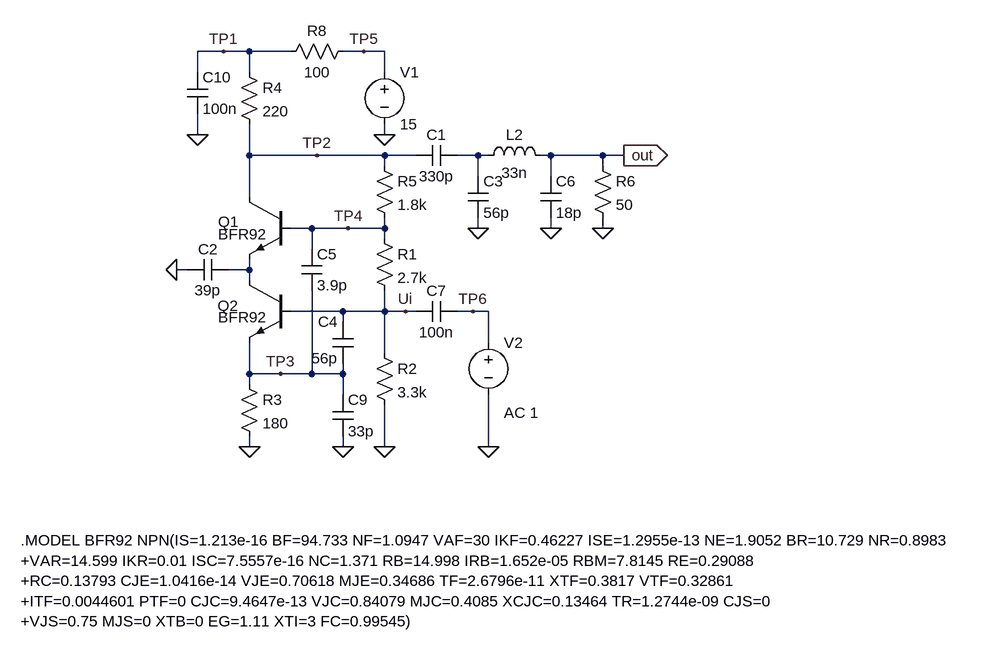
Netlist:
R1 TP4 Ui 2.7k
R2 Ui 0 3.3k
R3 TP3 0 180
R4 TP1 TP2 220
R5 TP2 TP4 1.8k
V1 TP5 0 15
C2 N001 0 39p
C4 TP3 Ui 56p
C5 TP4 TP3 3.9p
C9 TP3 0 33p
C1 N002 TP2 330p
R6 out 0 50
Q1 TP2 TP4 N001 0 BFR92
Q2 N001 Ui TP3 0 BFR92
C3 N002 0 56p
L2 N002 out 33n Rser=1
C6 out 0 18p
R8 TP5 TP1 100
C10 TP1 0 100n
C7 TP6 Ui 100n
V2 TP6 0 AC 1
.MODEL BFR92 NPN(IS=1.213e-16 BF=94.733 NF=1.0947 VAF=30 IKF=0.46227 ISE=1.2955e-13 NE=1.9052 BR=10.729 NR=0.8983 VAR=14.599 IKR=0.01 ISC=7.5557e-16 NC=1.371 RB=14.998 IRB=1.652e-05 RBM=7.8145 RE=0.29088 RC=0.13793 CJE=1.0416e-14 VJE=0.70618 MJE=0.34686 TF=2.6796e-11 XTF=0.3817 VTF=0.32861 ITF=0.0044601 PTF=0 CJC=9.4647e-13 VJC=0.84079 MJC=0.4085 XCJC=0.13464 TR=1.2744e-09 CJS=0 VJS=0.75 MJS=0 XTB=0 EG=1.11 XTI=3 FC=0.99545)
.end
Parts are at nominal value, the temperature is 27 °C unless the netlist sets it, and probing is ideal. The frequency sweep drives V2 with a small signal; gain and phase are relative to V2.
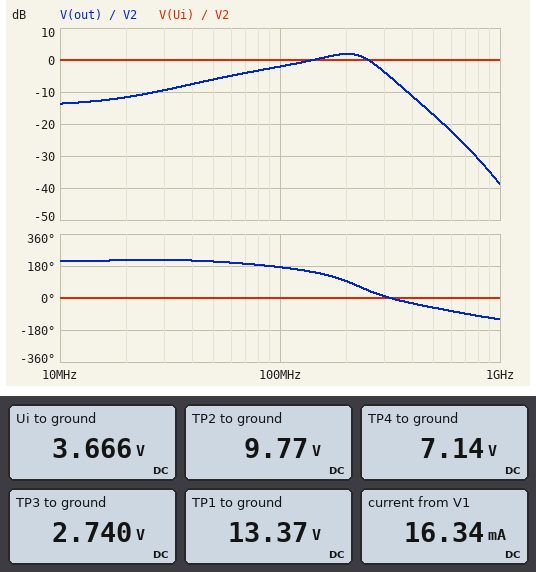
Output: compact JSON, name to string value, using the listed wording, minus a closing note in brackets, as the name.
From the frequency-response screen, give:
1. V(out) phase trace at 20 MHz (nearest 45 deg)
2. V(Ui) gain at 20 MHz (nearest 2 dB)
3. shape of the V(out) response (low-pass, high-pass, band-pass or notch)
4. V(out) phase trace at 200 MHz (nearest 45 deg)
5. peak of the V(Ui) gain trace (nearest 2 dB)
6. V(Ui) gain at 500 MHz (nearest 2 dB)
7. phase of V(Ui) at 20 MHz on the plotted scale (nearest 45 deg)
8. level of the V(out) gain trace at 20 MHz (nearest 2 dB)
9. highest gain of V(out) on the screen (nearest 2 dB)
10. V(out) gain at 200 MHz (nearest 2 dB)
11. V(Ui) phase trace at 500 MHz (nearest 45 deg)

{"V(out) phase trace at 20 MHz": "225 deg", "V(Ui) gain at 20 MHz": "0 dB", "shape of the V(out) response": "band-pass", "V(out) phase trace at 200 MHz": "90 deg", "peak of the V(Ui) gain trace": "0 dB", "V(Ui) gain at 500 MHz": "0 dB", "phase of V(Ui) at 20 MHz on the plotted scale": "0 deg", "level of the V(out) gain trace at 20 MHz": "-12 dB", "highest gain of V(out) on the screen": "2 dB", "V(out) gain at 200 MHz": "2 dB", "V(Ui) phase trace at 500 MHz": "0 deg"}
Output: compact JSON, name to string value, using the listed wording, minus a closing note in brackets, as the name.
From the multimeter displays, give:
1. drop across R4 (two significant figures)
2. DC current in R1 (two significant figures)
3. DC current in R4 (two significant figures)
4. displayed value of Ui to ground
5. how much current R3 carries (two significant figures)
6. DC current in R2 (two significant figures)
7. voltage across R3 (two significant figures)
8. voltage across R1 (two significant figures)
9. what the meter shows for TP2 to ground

{"drop across R4": "3.6 V", "DC current in R1": "1.3 mA", "DC current in R4": "16 mA", "displayed value of Ui to ground": "3.666 V", "how much current R3 carries": "15 mA", "DC current in R2": "1.1 mA", "voltage across R3": "2.7 V", "voltage across R1": "3.5 V", "what the meter shows for TP2 to ground": "9.77 V"}
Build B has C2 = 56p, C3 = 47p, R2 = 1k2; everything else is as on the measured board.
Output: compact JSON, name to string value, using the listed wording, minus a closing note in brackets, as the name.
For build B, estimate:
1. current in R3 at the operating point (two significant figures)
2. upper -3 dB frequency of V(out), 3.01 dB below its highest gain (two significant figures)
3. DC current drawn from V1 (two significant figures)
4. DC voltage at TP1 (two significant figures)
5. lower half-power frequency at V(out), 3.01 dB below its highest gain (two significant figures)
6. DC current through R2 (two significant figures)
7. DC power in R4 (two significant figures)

{"current in R3 at the operating point": "8.1 mA", "upper -3 dB frequency of V(out), 3.01 dB below its highest gain": "260 MHz", "DC current drawn from V1": "10 mA", "DC voltage at TP1": "14 V", "lower half-power frequency at V(out), 3.01 dB below its highest gain": "110 MHz", "DC current through R2": "2.0 mA", "DC power in R4": "22 mW"}
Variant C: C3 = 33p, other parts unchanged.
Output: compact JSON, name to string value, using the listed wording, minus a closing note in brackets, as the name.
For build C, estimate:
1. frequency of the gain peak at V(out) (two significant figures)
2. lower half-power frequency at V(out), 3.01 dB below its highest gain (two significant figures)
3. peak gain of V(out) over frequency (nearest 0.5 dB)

{"frequency of the gain peak at V(out)": "230 MHz", "lower half-power frequency at V(out), 3.01 dB below its highest gain": "150 MHz", "peak gain of V(out) over frequency": "5.5 dB"}
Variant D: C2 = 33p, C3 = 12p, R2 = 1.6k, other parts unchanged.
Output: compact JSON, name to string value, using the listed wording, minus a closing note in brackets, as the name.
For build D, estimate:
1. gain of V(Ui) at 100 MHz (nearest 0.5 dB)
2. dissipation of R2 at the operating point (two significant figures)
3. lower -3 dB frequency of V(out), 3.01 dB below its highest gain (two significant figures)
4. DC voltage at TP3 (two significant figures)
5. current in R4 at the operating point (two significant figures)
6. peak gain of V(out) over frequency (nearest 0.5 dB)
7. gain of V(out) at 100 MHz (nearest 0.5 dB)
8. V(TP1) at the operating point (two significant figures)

{"gain of V(Ui) at 100 MHz": "0 dB", "dissipation of R2 at the operating point": "4.7 mW", "lower -3 dB frequency of V(out), 3.01 dB below its highest gain": "200 MHz", "DC voltage at TP3": "1.8 V", "current in R4 at the operating point": "12 mA", "peak gain of V(out) over frequency": "9.0 dB", "gain of V(out) at 100 MHz": "0.5 dB", "V(TP1) at the operating point": "14 V"}
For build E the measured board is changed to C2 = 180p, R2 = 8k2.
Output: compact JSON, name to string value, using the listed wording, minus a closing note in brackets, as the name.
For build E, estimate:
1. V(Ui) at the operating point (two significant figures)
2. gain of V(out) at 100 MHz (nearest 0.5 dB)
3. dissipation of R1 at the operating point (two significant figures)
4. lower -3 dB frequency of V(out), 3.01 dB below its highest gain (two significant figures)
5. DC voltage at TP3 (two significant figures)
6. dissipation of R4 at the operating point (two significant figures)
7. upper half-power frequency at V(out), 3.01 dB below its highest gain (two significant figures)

{"V(Ui) at the operating point": "4.5 V", "gain of V(out) at 100 MHz": "2.0 dB", "dissipation of R1 at the operating point": "1.7 mW", "lower -3 dB frequency of V(out), 3.01 dB below its highest gain": "86 MHz", "DC voltage at TP3": "3.6 V", "dissipation of R4 at the operating point": "91 mW", "upper half-power frequency at V(out), 3.01 dB below its highest gain": "260 MHz"}
